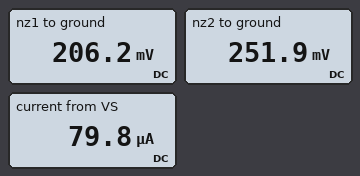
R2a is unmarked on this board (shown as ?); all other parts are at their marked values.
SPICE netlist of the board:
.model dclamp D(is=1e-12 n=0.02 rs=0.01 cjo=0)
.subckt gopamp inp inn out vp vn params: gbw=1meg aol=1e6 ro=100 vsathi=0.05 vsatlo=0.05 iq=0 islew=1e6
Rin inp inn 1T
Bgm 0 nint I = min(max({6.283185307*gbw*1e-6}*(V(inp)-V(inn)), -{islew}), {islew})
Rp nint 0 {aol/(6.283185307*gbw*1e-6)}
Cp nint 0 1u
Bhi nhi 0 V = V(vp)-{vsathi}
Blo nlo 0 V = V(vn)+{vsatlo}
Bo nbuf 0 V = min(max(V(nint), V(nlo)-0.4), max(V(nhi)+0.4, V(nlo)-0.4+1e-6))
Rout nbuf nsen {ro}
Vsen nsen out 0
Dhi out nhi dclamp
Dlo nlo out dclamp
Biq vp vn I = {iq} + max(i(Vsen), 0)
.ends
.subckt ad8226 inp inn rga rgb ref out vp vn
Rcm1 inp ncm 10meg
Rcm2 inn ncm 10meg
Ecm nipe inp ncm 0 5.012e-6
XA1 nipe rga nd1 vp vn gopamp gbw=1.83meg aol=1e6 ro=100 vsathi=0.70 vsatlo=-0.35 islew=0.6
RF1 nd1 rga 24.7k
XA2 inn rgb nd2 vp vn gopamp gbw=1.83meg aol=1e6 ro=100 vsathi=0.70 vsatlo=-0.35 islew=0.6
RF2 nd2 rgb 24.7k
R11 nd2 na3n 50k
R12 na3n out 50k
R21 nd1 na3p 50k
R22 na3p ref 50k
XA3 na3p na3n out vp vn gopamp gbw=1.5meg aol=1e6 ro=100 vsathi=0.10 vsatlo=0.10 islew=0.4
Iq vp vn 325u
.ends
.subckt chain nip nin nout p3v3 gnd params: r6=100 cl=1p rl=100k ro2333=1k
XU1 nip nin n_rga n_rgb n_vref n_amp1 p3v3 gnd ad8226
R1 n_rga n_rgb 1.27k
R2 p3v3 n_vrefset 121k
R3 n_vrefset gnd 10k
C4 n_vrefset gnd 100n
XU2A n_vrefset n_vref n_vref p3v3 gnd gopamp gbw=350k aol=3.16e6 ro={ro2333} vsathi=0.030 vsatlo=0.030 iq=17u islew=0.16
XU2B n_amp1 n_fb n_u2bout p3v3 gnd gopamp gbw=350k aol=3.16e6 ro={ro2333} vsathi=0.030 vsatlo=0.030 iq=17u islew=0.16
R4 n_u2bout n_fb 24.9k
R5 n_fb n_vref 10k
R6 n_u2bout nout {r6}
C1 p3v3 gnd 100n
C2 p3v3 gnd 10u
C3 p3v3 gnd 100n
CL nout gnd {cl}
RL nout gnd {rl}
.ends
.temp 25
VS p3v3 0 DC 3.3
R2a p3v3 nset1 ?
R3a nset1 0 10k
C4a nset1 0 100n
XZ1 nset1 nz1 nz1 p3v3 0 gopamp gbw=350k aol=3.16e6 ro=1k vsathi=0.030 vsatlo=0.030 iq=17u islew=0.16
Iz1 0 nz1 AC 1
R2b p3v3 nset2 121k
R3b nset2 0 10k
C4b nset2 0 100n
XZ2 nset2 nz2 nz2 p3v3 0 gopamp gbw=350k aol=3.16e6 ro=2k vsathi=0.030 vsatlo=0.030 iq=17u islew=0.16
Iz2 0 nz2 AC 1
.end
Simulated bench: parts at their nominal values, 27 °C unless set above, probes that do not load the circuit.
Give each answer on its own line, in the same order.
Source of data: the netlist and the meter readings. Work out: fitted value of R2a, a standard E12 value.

150 kΩ
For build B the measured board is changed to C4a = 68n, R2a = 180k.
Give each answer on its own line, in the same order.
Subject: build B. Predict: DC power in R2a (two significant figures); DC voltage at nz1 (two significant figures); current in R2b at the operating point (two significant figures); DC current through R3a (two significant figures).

54 µW
170 mV
25 µA
17 µA
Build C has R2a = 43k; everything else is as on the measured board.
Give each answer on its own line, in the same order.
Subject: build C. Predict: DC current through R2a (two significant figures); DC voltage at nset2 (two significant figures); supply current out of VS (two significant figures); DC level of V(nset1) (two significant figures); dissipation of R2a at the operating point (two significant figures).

62 µA
250 mV
120 µA
620 mV
170 µW
